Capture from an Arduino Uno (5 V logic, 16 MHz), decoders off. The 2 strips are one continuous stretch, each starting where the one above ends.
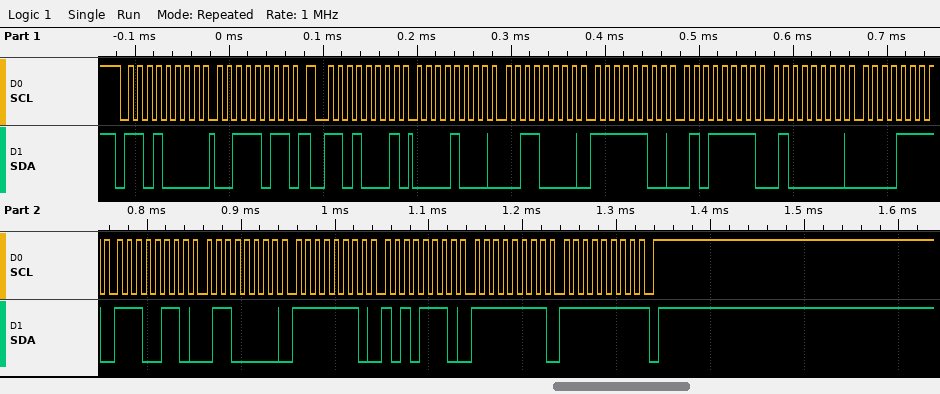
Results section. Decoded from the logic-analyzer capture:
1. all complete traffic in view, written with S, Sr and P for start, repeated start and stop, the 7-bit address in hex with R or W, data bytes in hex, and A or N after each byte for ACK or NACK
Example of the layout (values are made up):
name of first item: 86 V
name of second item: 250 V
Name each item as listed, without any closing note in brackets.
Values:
all complete traffic in view, written with S, Sr and P for start, repeated start and stop, the 7-bit address in hex with R or W, data bytes in hex, and A or N after each byte for ACK or NACK: S 68W A 3B A Sr 68R A 08 A 30 A FC A 5F A 40 A 0F A E6 A 60 A FE A AE A FF A FF N P
